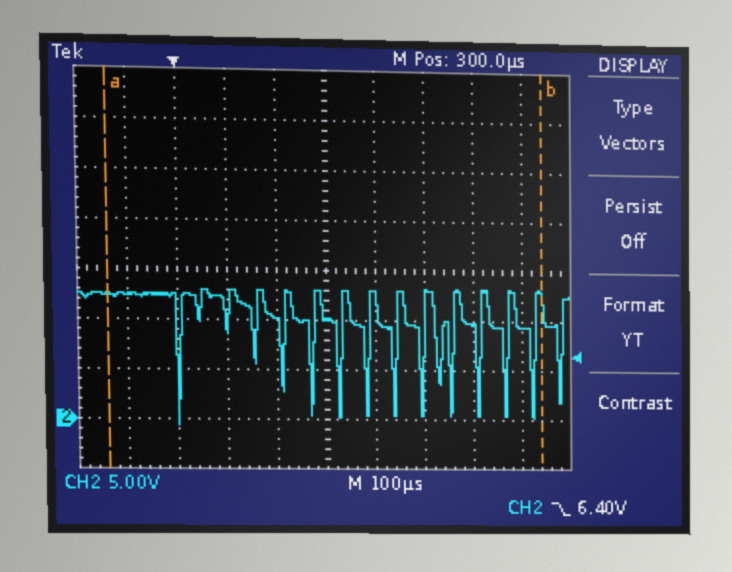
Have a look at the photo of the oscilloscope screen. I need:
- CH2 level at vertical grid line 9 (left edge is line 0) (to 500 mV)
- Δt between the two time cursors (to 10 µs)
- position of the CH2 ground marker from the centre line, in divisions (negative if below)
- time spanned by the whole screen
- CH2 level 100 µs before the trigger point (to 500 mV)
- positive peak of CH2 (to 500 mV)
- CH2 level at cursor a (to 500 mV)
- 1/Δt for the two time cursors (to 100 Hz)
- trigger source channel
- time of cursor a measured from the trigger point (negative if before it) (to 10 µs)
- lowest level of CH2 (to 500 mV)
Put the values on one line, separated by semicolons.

9.5 V; 880 µs; -3.0 div; 1 ms; 12.5 V; 13.0 V; 12.5 V; 1.1 kHz; CH2; -140 µs; -500 mV
